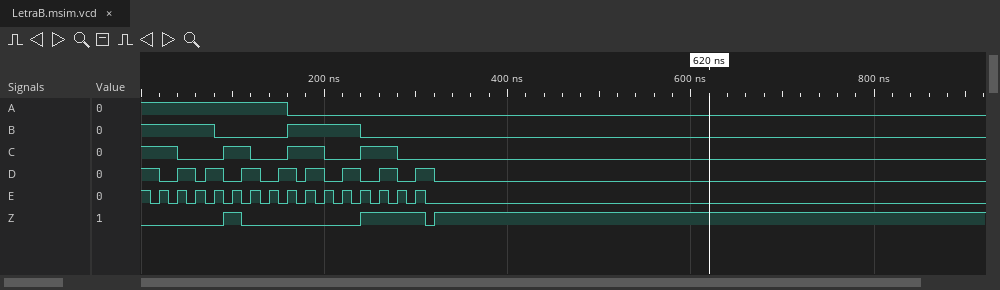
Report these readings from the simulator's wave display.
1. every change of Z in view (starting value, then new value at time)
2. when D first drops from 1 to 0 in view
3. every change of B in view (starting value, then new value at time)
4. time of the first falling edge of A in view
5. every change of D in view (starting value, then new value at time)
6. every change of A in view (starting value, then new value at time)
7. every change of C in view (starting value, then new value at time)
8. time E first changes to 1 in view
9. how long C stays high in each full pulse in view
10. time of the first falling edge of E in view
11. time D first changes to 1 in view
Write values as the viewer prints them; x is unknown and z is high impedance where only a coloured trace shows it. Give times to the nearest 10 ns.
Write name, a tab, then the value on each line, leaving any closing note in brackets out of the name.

every change of Z in view	0, 1 at 90 ns, 0 at 110 ns, 1 at 240 ns, 0 at 310 ns, 1 at 320 ns
when D first drops from 1 to 0 in view	20 ns
every change of B in view	1, 0 at 80 ns, 1 at 160 ns, 0 at 240 ns
time of the first falling edge of A in view	160 ns
every change of D in view	1, 0 at 20 ns, 1 at 40 ns, 0 at 60 ns, 1 at 70 ns, 0 at 90 ns, 1 at 110 ns, 0 at 130 ns, 1 at 150 ns, 0 at 170 ns, 1 at 180 ns, 0 at 200 ns, 1 at 220 ns, 0 at 240 ns, 1 at 260 ns, 0 at 280 ns, 1 at 300 ns, 0 at 320 ns
every change of A in view	1, 0 at 160 ns
every change of C in view	1, 0 at 40 ns, 1 at 90 ns, 0 at 120 ns, 1 at 160 ns, 0 at 200 ns, 1 at 240 ns, 0 at 280 ns
time E first changes to 1 in view	20 ns
how long C stays high in each full pulse in view	30 ns, 40 ns, 40 ns
time of the first falling edge of E in view	10 ns
time D first changes to 1 in view	40 ns
